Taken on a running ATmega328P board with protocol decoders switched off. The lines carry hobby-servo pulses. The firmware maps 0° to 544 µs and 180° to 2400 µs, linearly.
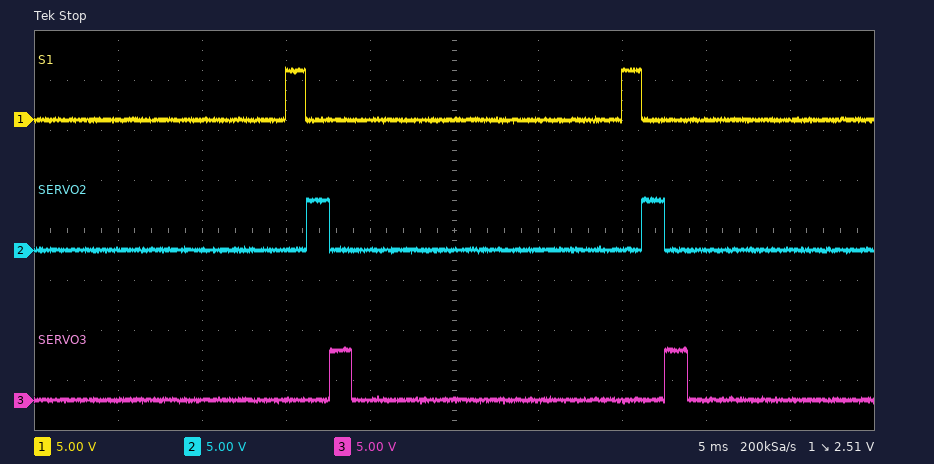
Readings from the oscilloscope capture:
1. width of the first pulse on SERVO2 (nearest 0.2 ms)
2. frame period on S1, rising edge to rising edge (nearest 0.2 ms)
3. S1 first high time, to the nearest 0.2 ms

1.4 ms
20.0 ms
1.2 ms
